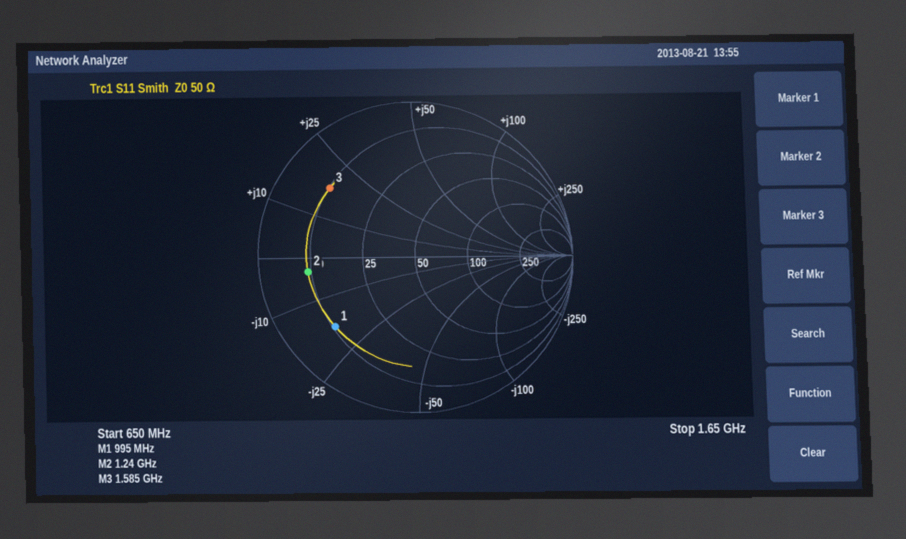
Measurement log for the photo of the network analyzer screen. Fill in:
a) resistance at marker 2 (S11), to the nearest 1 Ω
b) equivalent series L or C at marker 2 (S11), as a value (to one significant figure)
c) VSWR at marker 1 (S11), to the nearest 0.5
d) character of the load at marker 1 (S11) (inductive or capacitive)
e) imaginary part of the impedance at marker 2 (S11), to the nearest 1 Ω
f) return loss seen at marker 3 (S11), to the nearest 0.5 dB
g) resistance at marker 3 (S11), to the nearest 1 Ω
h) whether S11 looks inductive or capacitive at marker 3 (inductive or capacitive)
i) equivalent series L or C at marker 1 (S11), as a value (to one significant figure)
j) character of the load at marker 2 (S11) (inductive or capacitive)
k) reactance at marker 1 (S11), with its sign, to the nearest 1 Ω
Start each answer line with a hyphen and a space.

- 9 Ω
- 40 pF
- 5.5
- capacitive
- -3 Ω
- 3.0 dB
- 10 Ω
- inductive
- 9 pF
- capacitive
- -18 Ω
